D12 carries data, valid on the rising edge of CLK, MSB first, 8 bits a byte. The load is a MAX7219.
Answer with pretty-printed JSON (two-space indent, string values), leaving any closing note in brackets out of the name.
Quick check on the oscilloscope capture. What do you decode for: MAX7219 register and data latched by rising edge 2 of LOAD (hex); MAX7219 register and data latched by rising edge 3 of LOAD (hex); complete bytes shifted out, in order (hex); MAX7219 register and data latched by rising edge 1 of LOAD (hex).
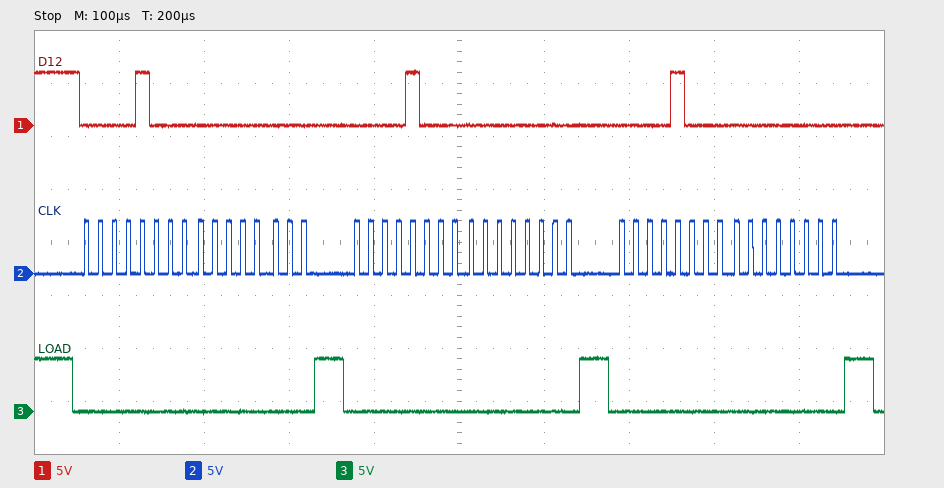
{
  "MAX7219 register and data latched by rising edge 2 of LOAD": "register 0x8, data 0x00",
  "MAX7219 register and data latched by rising edge 3 of LOAD": "register 0x8, data 0x00",
  "complete bytes shifted out, in order": "08 00 08 00 08 00",
  "MAX7219 register and data latched by rising edge 1 of LOAD": "register 0x8, data 0x00"
}
